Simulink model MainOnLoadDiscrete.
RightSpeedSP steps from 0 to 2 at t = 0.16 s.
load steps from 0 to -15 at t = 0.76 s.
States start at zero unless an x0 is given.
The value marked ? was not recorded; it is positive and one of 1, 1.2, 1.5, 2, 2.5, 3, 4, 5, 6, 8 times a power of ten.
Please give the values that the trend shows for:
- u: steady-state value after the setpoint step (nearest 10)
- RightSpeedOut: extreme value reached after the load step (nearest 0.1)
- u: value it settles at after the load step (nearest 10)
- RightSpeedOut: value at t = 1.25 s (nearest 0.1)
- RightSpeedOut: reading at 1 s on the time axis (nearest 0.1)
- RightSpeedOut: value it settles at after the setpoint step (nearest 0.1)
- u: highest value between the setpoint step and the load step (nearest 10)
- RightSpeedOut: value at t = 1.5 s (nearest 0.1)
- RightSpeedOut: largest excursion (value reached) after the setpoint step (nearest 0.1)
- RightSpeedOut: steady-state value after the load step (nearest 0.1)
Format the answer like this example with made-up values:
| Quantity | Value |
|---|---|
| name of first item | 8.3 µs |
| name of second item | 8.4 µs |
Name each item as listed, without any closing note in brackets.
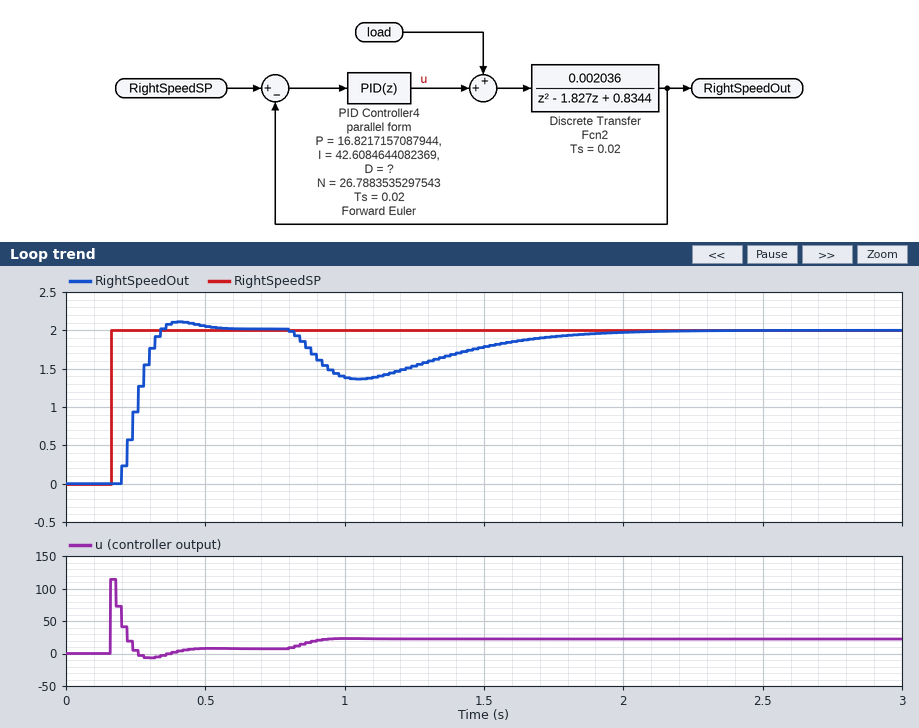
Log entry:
| Quantity | Value |
|---|---|
| u: steady-state value after the setpoint step | 10 |
| RightSpeedOut: extreme value reached after the load step | 1.4 |
| u: value it settles at after the load step | 20 |
| RightSpeedOut: value at t = 1.25 s | 1.5 |
| RightSpeedOut: reading at 1 s on the time axis | 1.4 |
| RightSpeedOut: value it settles at after the setpoint step | 2.0 |
| u: highest value between the setpoint step and the load step | 110 |
| RightSpeedOut: value at t = 1.5 s | 1.8 |
| RightSpeedOut: largest excursion (value reached) after the setpoint step | 2.1 |
| RightSpeedOut: steady-state value after the load step | 2.0 |
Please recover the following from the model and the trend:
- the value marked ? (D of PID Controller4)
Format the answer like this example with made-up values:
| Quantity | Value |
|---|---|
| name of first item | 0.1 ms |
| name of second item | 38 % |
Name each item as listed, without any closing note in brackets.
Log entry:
| Quantity | Value |
|---|---|
| the value marked ? | 1.5 |
